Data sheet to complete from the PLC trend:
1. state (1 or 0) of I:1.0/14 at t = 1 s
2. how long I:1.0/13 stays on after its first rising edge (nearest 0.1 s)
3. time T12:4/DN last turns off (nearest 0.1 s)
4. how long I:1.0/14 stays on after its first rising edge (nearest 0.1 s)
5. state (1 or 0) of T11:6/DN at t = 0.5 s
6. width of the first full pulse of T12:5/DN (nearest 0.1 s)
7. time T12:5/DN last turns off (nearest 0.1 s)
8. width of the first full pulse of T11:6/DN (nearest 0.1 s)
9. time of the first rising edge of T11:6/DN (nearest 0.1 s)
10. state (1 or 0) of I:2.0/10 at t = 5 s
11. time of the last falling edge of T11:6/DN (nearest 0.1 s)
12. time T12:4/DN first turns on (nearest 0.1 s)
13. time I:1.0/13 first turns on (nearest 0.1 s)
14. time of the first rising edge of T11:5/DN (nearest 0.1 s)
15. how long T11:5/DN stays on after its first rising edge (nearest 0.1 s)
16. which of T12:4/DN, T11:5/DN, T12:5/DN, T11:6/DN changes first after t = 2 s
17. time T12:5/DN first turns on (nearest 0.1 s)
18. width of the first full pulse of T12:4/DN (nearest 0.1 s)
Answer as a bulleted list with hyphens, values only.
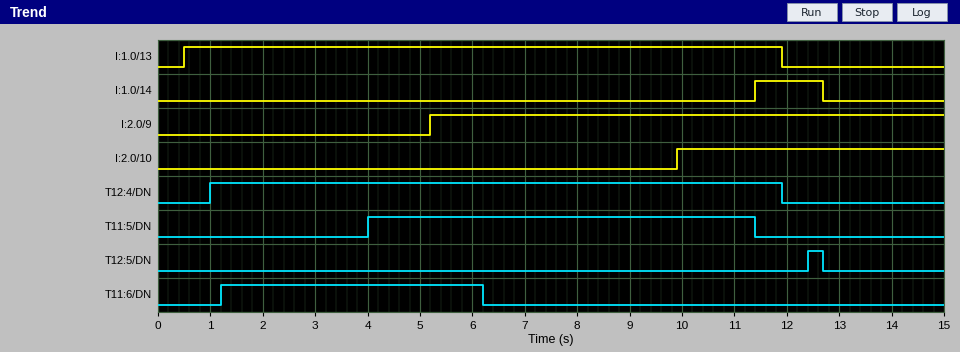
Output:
- 0
- 11.4 s
- 11.9 s
- 1.3 s
- 0
- 0.3 s
- 12.7 s
- 5.0 s
- 1.2 s
- 0
- 6.2 s
- 1.0 s
- 0.5 s
- 4.0 s
- 7.4 s
- T11:5/DN
- 12.4 s
- 10.9 s
